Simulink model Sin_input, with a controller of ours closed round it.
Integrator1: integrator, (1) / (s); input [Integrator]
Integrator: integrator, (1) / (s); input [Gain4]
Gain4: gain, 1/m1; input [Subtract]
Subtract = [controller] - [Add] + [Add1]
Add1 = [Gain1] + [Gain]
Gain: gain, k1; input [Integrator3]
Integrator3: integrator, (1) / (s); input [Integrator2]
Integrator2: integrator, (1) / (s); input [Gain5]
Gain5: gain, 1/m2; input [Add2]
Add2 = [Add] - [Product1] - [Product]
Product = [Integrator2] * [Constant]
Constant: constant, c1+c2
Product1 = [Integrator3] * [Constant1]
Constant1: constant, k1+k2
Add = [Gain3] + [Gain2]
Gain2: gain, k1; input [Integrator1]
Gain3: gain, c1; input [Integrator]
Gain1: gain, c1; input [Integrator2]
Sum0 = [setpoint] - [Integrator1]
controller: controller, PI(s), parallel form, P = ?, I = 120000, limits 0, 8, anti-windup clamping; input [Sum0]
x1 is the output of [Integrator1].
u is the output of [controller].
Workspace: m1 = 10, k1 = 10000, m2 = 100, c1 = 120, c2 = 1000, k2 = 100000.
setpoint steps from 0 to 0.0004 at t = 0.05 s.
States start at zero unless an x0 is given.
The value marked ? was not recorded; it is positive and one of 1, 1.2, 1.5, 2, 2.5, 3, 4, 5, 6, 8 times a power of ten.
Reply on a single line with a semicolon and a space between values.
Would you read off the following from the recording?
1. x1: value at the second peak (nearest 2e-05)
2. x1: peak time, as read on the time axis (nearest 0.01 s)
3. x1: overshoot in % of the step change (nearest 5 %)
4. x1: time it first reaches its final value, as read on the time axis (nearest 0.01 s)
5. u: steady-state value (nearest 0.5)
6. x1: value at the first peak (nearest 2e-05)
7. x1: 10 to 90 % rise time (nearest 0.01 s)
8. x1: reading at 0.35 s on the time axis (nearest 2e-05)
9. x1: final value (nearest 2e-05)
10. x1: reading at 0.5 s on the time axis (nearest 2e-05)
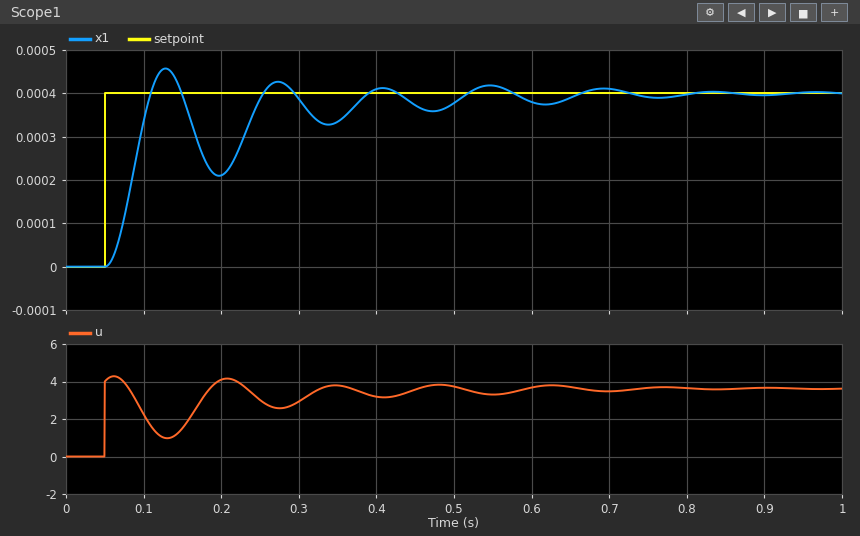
0.00042; 0.13 s; 15 %; 0.11 s; 3.5; 0.00046; 0.04 s; 0.00034; 0.00040; 0.00038
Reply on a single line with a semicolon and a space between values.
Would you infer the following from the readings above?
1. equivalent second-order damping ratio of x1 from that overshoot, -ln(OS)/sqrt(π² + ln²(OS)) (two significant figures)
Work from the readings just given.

0.52
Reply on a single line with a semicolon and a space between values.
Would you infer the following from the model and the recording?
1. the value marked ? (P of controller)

10000
